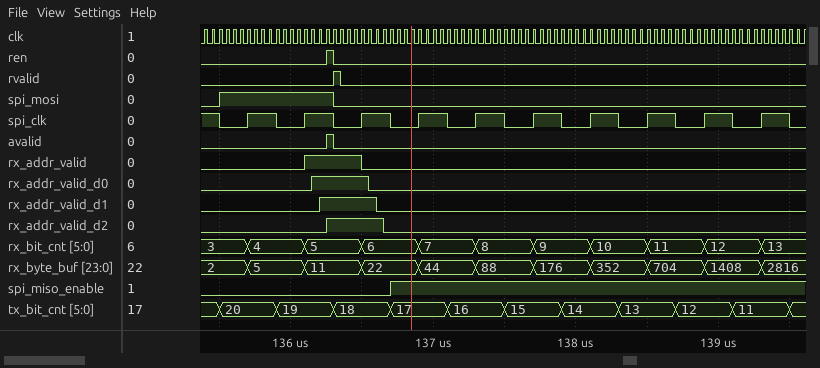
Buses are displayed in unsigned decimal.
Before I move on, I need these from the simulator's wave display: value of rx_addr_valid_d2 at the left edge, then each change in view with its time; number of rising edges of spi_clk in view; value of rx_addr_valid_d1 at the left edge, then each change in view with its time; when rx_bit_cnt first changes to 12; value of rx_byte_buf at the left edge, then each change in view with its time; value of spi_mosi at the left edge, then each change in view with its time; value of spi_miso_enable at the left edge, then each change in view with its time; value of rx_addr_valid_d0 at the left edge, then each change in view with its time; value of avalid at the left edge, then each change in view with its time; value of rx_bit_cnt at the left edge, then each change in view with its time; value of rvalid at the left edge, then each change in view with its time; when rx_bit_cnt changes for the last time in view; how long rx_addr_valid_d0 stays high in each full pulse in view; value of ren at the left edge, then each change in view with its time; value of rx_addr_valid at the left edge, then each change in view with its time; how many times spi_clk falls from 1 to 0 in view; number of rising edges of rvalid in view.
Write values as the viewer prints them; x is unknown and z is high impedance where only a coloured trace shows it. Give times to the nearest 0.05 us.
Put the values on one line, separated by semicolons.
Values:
0, 1 at 136.25 us, 0 at 136.65 us; 10; 0, 1 at 136.2 us, 0 at 136.6 us; 138.9 us; 2, 5 at 135.7 us, 11 at 136.1 us, 22 at 136.5 us, 44 at 136.9 us, 88 at 137.3 us, 176 at 137.7 us, 352 at 138.1 us, 704 at 138.5 us, 1408 at 138.9 us, 2816 at 139.3 us; 0, 1 at 135.5 us, 0 at 136.3 us; 0, 1 at 136.7 us; 0, 1 at 136.15 us, 0 at 136.55 us; 0, 1 at 136.25 us, 0 at 136.3 us; 3, 4 at 135.7 us, 5 at 136.1 us, 6 at 136.5 us, 7 at 136.9 us, 8 at 137.3 us, 9 at 137.7 us, 10 at 138.1 us, 11 at 138.5 us, 12 at 138.9 us, 13 at 139.3 us; 0, 1 at 136.3 us, 0 at 136.35 us; 139.3 us; 0.4 us; 0, 1 at 136.25 us, 0 at 136.3 us; 0, 1 at 136.1 us, 0 at 136.5 us; 11; 1
